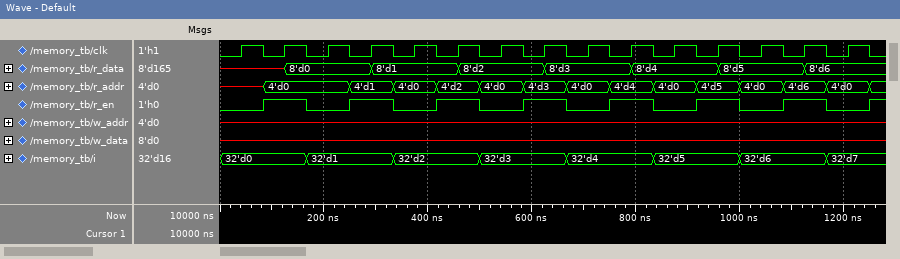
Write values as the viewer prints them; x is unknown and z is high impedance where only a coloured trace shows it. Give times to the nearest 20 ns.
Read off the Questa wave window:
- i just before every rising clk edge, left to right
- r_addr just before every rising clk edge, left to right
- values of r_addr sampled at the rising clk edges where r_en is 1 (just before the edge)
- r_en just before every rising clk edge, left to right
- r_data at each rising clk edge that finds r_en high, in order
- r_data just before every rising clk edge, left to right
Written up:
32'd0, 32'd0, 32'd1, 32'd1, 32'd2, 32'd2, 32'd3, 32'd3, 32'd4, 32'd4, 32'd5, 32'd5, 32'd6, 32'd6, 32'd7
x, 4'd0, 4'd0, 4'd1, 4'd0, 4'd2, 4'd0, 4'd3, 4'd0, 4'd4, 4'd0, 4'd5, 4'd0, 4'd6, 4'd0
4'd0, 4'd1, 4'd2, 4'd3, 4'd4, 4'd5, 4'd6
0 1 0 1 0 1 0 1 0 1 0 1 0 1 0
x, 8'd0, 8'd1, 8'd2, 8'd3, 8'd4, 8'd5
x, x, 8'd0, 8'd0, 8'd1, 8'd1, 8'd2, 8'd2, 8'd3, 8'd3, 8'd4, 8'd4, 8'd5, 8'd5, 8'd6
